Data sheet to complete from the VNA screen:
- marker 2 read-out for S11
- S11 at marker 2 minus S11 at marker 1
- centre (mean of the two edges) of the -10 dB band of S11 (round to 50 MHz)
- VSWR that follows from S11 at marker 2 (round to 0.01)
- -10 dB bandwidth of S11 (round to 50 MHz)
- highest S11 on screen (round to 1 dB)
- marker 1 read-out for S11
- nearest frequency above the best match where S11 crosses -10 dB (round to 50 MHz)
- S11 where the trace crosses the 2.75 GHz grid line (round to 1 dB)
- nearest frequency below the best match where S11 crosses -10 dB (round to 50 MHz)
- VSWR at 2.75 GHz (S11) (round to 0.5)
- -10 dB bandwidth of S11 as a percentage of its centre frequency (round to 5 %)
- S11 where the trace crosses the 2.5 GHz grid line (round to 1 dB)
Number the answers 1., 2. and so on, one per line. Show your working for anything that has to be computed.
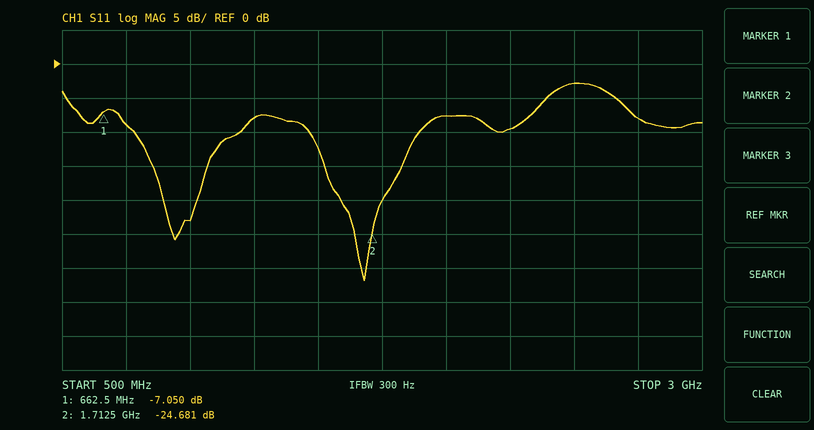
1. -24.681 dB
2. -24.681 − (-7.05) = -17.631 dB
3. 1.70 GHz
4. (1 + 0.0583)/(1 − 0.0583) ≈ 1.12
5. 1.90 GHz − 1.45 GHz = 450 MHz
6. -3 dB
7. -7.050 dB
8. 1.90 GHz
9. -8 dB
10. 1.45 GHz
11. |Γ| = 10^(-8/20) = 0.3981; VSWR = (1 + 0.3981)/(1 − 0.3981) ≈ 2.32, so 2.5 to the nearest 0.5
12. 450 MHz / 1.675 GHz ≈ 26.9 %, so 25 % to the nearest 5 %
13. -3 dB
